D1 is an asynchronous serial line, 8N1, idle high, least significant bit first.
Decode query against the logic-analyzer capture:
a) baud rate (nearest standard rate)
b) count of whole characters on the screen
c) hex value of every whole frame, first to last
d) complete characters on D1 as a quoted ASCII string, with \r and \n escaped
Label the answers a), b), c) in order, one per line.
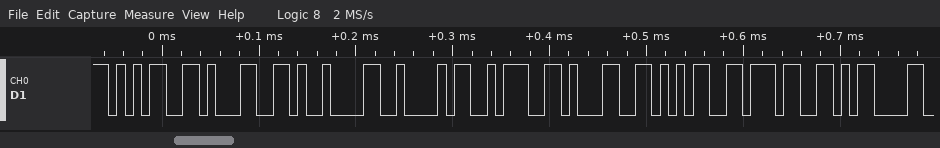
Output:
a) 115200 baud
b) 9
c) 35 31 09 42 3A 31 35 37 0D
d) "51\tB:157\r"
